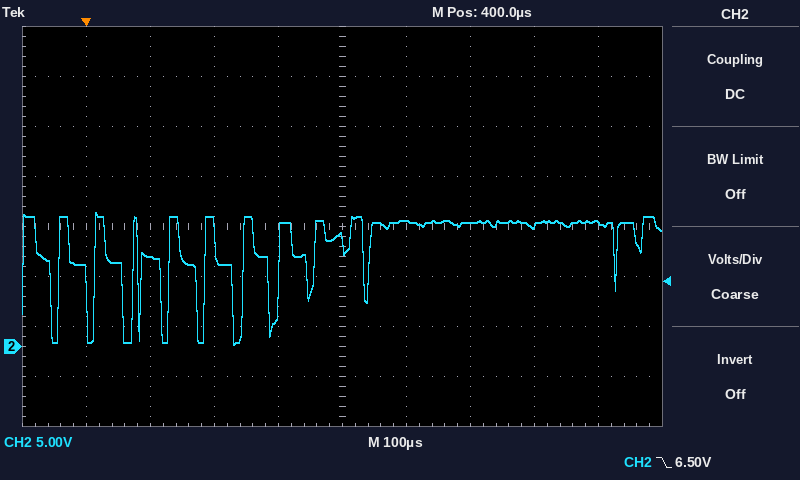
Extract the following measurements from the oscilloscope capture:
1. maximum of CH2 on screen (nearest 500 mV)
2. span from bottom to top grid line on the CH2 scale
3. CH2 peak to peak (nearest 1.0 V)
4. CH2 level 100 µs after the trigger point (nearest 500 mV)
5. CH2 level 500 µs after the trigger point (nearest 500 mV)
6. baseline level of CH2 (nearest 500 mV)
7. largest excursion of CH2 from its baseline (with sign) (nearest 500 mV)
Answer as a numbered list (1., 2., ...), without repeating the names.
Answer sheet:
1. 13.5 V
2. 40 V
3. 13.0 V
4. 9.0 V
5. 12.5 V
6. 12.5 V
7. -12.0 V
